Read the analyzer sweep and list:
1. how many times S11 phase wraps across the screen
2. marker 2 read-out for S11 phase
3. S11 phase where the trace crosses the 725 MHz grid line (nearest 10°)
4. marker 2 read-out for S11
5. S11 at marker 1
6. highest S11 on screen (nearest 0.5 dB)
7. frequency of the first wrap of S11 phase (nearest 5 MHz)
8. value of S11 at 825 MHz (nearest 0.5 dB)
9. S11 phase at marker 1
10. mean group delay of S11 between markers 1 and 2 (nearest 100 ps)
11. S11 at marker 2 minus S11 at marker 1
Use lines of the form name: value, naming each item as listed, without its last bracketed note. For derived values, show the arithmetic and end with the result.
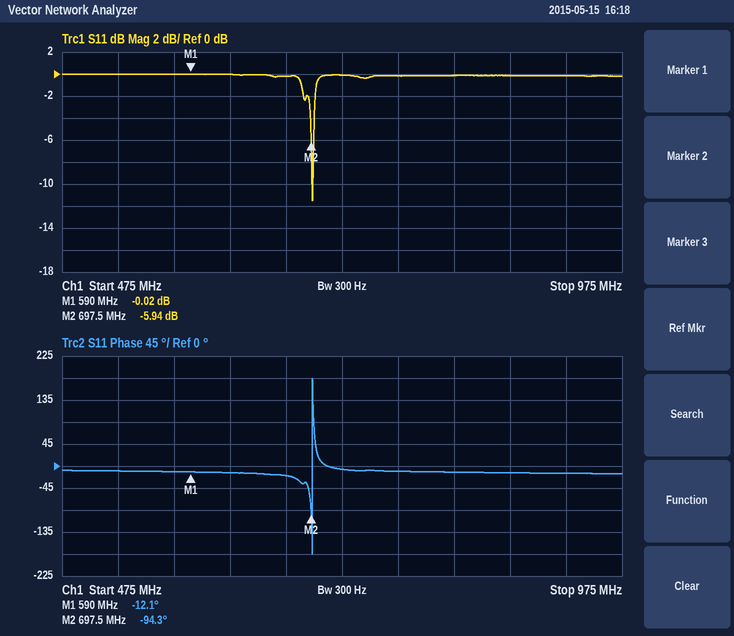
how many times S11 phase wraps across the screen: 1
marker 2 read-out for S11 phase: -94.3°
S11 phase where the trace crosses the 725 MHz grid line: -10°
marker 2 read-out for S11: -5.94 dB
S11 at marker 1: -0.02 dB
highest S11 on screen: 0.0 dB
frequency of the first wrap of S11 phase: 700 MHz
value of S11 at 825 MHz: 0.0 dB
S11 phase at marker 1: -12.1°
mean group delay of S11 between markers 1 and 2: −(-94.3° − (-12.1°))/(360° × 107.5 MHz) ≈ 2.1 ns
S11 at marker 2 minus S11 at marker 1: -5.94 − (-0.02) = -5.92 dB
